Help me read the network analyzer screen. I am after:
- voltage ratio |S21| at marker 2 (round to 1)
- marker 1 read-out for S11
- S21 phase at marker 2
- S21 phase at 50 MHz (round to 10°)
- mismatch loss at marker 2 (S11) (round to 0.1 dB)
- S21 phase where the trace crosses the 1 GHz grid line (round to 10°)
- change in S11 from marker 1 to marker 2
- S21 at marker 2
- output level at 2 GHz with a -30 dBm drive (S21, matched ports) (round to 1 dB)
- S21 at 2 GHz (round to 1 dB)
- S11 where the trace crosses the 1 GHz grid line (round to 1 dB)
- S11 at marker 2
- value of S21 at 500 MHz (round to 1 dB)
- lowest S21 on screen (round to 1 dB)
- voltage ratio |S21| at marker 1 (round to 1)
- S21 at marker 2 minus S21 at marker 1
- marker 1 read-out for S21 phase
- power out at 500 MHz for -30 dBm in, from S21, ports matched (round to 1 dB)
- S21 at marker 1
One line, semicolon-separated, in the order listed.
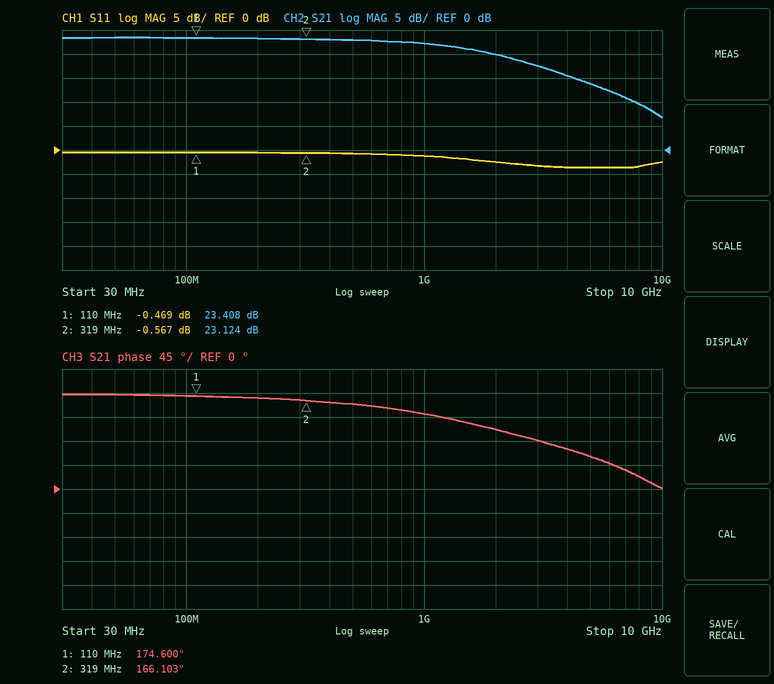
14; -0.469 dB; 166.103°; 180°; 9.1 dB; 140°; -0.098 dB; 23.124 dB; -10 dBm; 20 dB; -1 dB; -0.567 dB; 23 dB; 7 dB; 15; -0.284 dB; 174.600°; -7 dBm; 23.408 dB
